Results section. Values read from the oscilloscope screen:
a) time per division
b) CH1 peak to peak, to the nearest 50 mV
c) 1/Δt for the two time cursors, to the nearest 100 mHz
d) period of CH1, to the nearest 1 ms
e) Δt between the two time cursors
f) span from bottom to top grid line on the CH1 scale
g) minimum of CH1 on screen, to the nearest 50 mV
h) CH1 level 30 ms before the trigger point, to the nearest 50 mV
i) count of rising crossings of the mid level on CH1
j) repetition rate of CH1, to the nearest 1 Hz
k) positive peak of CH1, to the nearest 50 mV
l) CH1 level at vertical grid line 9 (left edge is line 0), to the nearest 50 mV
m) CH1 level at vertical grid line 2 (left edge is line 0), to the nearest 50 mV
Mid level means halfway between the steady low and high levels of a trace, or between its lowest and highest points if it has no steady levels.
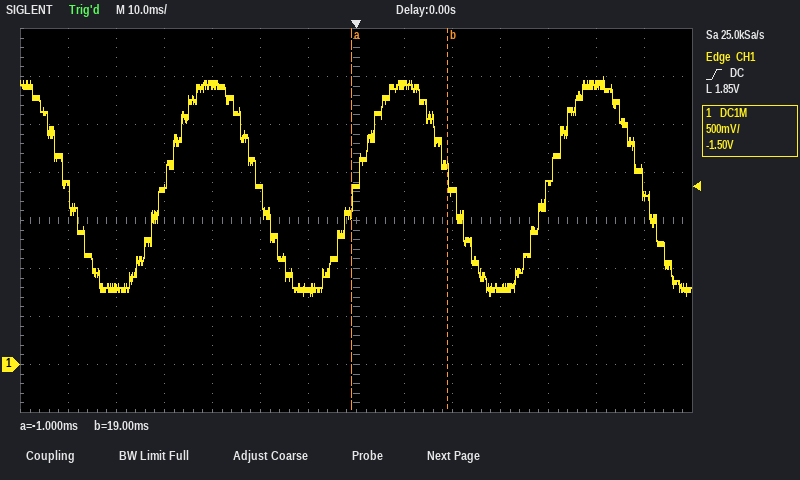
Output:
10 ms
2.30 V
50.0 Hz
40 ms
20 ms
4 V
700 mV
2.90 V
3
25 Hz
3.00 V
1.80 V
800 mV
